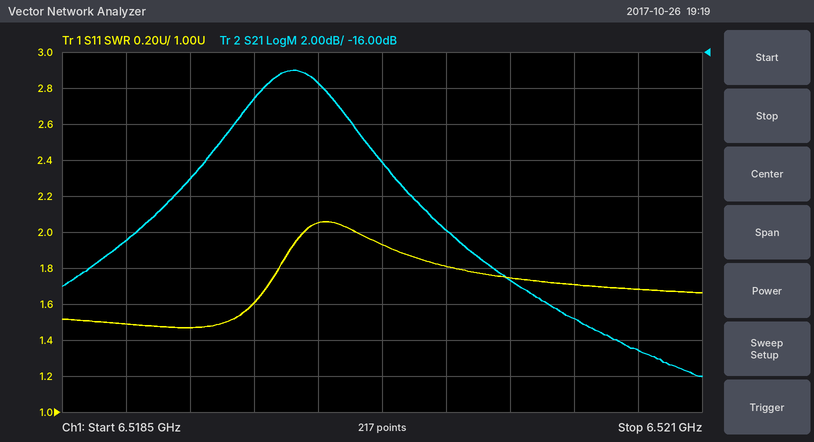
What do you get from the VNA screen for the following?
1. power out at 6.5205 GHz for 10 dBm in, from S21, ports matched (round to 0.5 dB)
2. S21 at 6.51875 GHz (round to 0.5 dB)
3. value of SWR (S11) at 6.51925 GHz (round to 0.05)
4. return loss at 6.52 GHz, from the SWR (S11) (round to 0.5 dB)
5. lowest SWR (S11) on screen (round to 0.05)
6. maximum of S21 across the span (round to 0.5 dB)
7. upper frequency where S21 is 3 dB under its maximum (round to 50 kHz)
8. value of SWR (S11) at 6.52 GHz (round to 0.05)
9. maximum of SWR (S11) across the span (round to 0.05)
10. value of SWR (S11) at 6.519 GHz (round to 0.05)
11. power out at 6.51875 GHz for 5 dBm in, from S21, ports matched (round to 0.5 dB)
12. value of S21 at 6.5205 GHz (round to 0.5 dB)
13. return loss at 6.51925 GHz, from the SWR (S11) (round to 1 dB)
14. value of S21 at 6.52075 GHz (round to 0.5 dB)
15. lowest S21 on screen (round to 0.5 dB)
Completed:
-21.0 dBm
-26.5 dB
1.60
11.0 dB
1.45
-17.0 dB
6.51965 GHz
1.80
2.05
1.45
-21.5 dBm
-31.0 dB
13 dB
-32.5 dB
-34.0 dB
